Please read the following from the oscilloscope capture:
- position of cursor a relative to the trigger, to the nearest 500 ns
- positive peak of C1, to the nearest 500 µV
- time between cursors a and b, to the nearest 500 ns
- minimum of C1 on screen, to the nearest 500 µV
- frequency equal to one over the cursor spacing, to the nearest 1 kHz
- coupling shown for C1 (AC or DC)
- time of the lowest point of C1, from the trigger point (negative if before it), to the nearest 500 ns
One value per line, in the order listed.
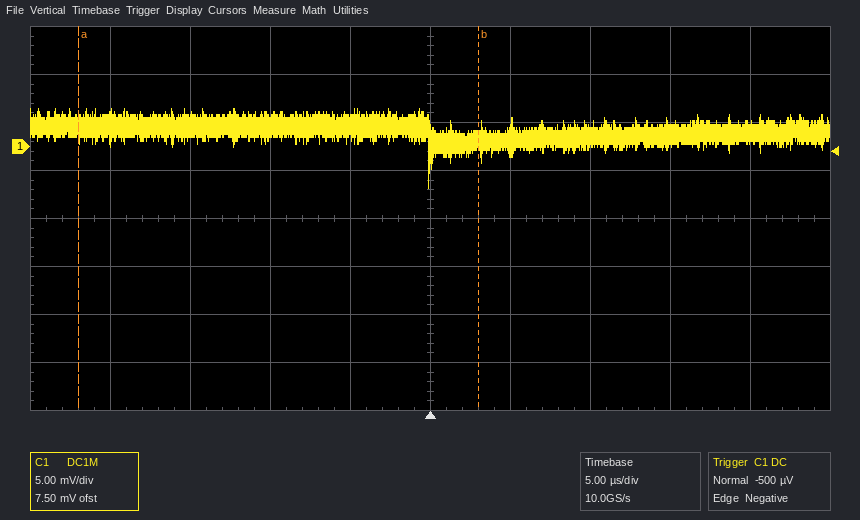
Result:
-22.0 µs
4.0 mV
25.0 µs
-4.5 mV
40 kHz
DC
0.0 µs
